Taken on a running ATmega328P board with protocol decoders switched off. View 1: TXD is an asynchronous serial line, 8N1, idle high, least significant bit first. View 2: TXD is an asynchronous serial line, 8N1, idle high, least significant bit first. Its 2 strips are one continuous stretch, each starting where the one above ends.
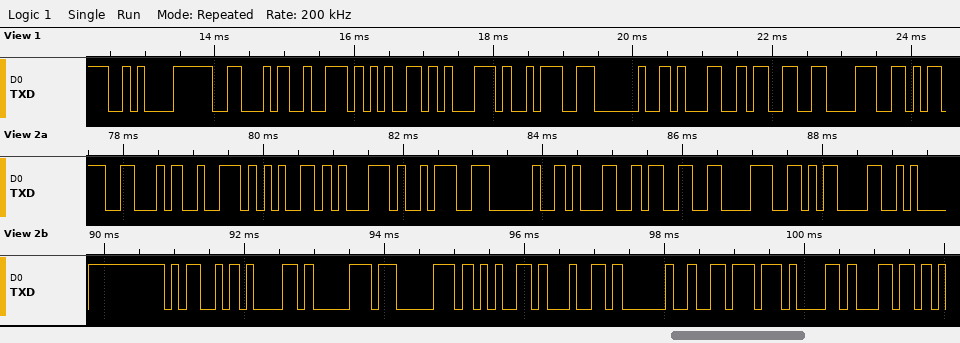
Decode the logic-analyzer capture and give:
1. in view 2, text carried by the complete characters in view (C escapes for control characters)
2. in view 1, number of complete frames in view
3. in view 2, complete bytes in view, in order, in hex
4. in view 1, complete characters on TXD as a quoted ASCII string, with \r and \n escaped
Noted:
"Freq: 138\r\nMapped val"
10
46 72 65 71 3A 20 31 33 38 0D 0A 4D 61 70 70 65 64 20 76 61 6C
"\nFreq: 138"
